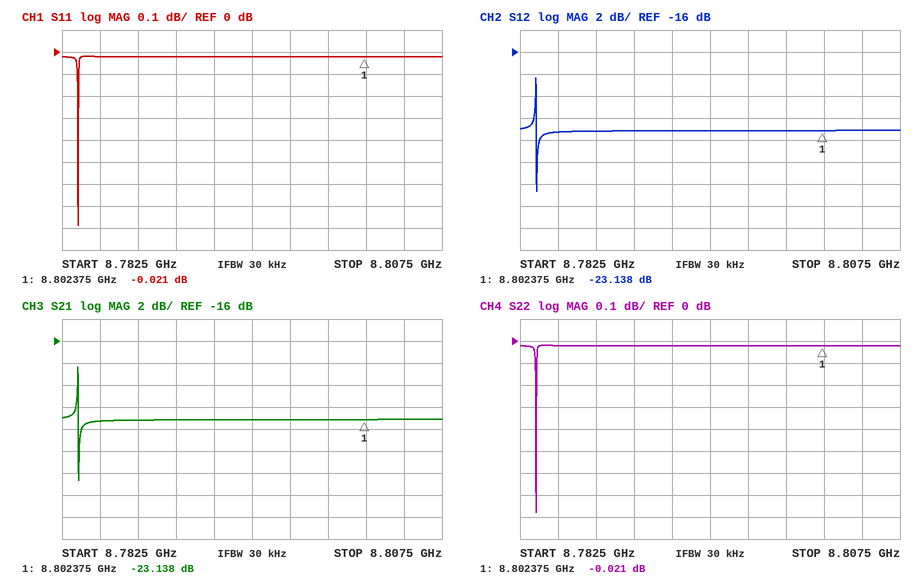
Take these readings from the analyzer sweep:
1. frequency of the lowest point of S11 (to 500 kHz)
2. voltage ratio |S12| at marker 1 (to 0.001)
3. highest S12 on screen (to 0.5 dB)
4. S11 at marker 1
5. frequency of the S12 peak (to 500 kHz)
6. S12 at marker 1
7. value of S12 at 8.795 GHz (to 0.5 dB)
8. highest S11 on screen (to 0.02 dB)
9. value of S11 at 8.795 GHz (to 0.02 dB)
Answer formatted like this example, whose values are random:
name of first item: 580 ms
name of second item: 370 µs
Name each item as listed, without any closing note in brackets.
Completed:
frequency of the lowest point of S11: 8.7835 GHz
voltage ratio |S12| at marker 1: 0.070
highest S12 on screen: -18.5 dB
S11 at marker 1: -0.021 dB
frequency of the S12 peak: 8.7835 GHz
S12 at marker 1: -23.138 dB
value of S12 at 8.795 GHz: -23.0 dB
highest S11 on screen: -0.02 dB
value of S11 at 8.795 GHz: -0.02 dB
